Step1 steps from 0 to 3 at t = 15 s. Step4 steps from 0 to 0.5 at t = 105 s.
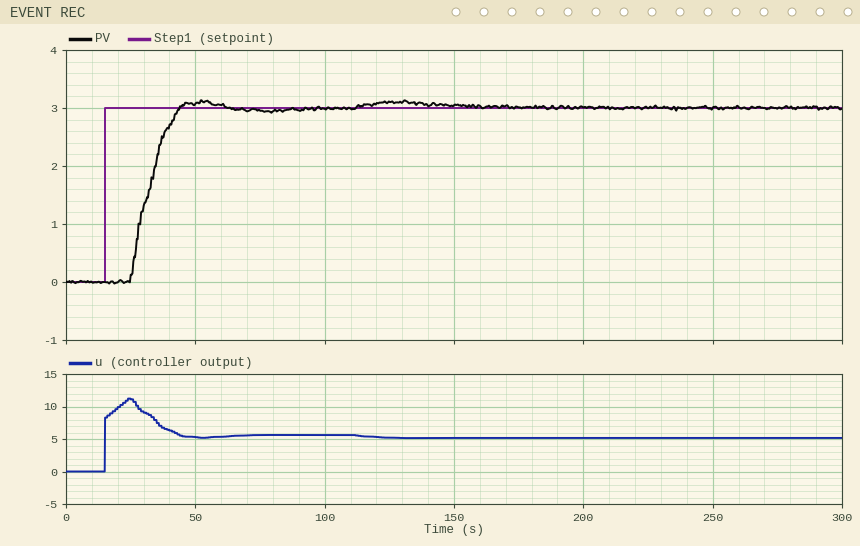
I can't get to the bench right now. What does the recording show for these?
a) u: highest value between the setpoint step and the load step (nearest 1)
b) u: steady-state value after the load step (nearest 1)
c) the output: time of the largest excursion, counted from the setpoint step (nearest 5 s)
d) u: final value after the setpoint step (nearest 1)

11
5
35 s
6
